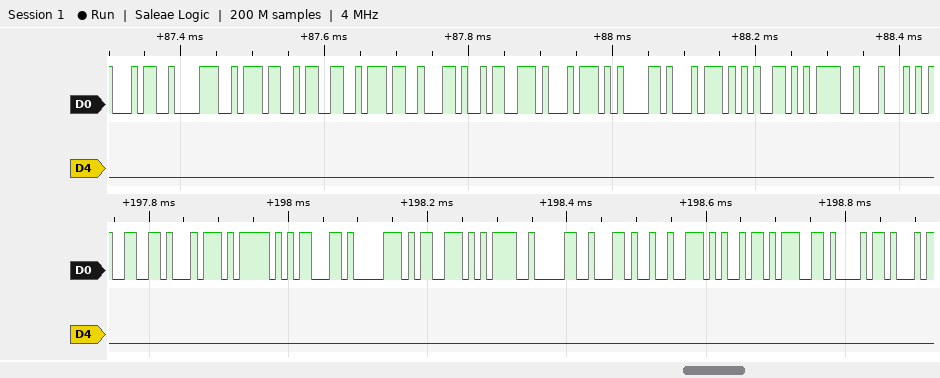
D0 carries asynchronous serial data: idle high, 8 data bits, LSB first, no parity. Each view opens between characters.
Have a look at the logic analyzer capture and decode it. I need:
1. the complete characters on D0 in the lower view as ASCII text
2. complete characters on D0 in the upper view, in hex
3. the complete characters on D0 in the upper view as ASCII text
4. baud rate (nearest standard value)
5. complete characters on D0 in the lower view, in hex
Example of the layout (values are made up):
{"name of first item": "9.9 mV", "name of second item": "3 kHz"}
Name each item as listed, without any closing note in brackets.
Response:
{"the complete characters on D0 in the lower view as ASCII text": "\"ft_cps=0,righ\"", "complete characters on D0 in the upper view, in hex": "34, 38, 37, 33, 37, 2C, 73, 74, 61, 74, 65, 3D, 44", "the complete characters on D0 in the upper view as ASCII text": "\"48737,state=D\"", "baud rate": "115200 baud", "complete characters on D0 in the lower view, in hex": "66, 74, 5F, 63, 70, 73, 3D, 30, 2C, 72, 69, 67, 68"}
